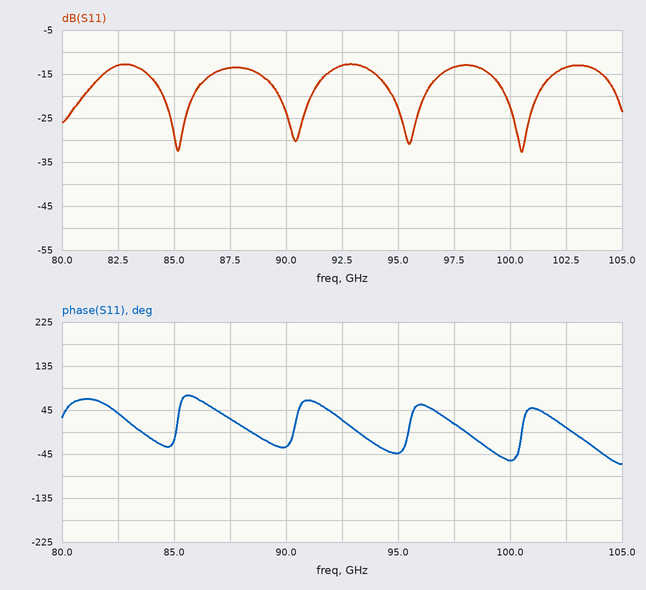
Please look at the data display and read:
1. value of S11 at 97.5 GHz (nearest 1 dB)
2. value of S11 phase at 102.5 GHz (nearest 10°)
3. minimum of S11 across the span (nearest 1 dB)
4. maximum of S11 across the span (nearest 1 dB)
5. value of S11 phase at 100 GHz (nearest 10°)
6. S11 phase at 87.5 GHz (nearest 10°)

-13 dB
10°
-33 dB
-13 dB
-60°
30°
